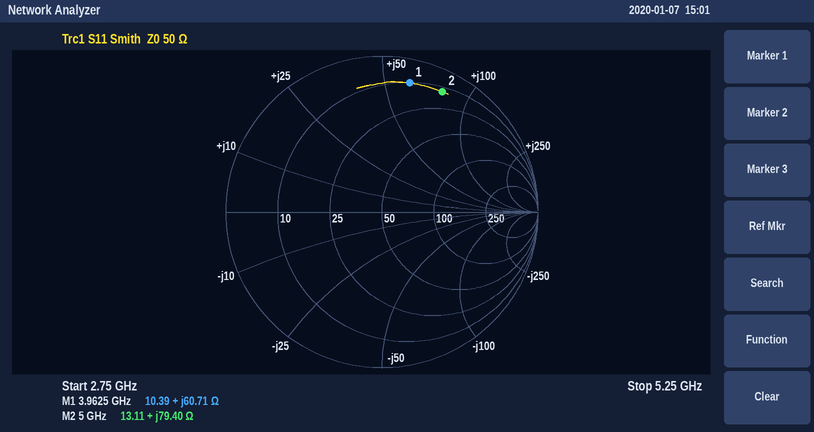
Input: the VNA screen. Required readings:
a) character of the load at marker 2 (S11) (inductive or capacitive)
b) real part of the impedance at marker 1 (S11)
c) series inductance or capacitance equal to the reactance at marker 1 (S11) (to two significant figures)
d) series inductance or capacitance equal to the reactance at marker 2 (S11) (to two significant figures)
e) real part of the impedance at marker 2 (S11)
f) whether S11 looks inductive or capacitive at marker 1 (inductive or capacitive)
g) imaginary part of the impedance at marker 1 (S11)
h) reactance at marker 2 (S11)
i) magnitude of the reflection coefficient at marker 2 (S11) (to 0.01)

inductive
10.39 Ω
2.4 nH
2.5 nH
13.11 Ω
inductive
+60.71 Ω
+79.40 Ω
0.86
